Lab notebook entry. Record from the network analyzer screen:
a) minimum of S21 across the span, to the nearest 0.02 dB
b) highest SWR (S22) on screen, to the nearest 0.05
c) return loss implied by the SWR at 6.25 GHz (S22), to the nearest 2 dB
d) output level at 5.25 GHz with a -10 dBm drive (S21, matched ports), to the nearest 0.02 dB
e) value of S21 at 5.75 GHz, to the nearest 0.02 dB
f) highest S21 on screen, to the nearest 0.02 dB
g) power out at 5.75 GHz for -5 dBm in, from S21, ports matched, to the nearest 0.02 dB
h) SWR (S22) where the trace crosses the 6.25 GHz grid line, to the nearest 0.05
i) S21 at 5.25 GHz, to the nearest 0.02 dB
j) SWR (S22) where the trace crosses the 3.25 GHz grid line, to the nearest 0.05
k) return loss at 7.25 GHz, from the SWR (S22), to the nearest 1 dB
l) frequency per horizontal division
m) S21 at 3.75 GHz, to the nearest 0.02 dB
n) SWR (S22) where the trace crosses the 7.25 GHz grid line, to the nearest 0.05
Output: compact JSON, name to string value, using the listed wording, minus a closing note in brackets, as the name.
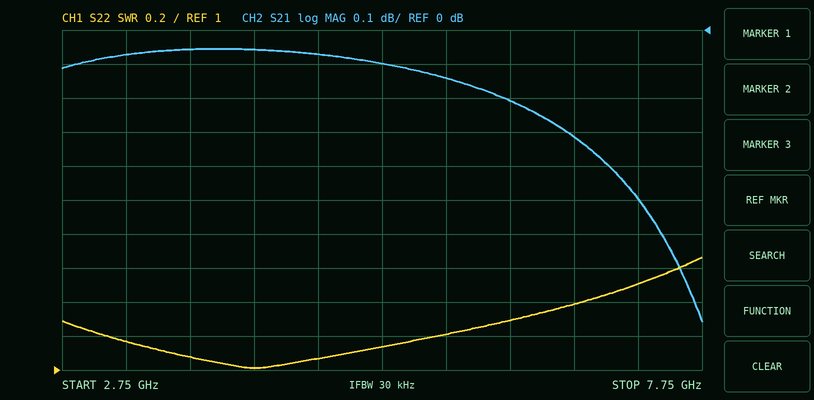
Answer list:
{"minimum of S21 across the span, to the nearest 0.02 dB": "-0.86 dB", "highest SWR (S22) on screen, to the nearest 0.05": "1.65", "return loss implied by the SWR at 6.25 GHz (S22), to the nearest 2 dB": "18 dB", "output level at 5.25 GHz with a -10 dBm drive (S21, matched ports), to the nearest 0.02 dB": "-10.10 dBm", "value of S21 at 5.75 GHz, to the nearest 0.02 dB": "-0.14 dB", "highest S21 on screen, to the nearest 0.02 dB": "-0.06 dB", "power out at 5.75 GHz for -5 dBm in, from S21, ports matched, to the nearest 0.02 dB": "-5.14 dBm", "SWR (S22) where the trace crosses the 6.25 GHz grid line, to the nearest 0.05": "1.30", "S21 at 5.25 GHz, to the nearest 0.02 dB": "-0.10 dB", "SWR (S22) where the trace crosses the 3.25 GHz grid line, to the nearest 0.05": "1.15", "return loss at 7.25 GHz, from the SWR (S22), to the nearest 1 dB": "14 dB", "frequency per horizontal division": "500 MHz", "S21 at 3.75 GHz, to the nearest 0.02 dB": "-0.06 dB", "SWR (S22) where the trace crosses the 7.25 GHz grid line, to the nearest 0.05": "1.50"}
